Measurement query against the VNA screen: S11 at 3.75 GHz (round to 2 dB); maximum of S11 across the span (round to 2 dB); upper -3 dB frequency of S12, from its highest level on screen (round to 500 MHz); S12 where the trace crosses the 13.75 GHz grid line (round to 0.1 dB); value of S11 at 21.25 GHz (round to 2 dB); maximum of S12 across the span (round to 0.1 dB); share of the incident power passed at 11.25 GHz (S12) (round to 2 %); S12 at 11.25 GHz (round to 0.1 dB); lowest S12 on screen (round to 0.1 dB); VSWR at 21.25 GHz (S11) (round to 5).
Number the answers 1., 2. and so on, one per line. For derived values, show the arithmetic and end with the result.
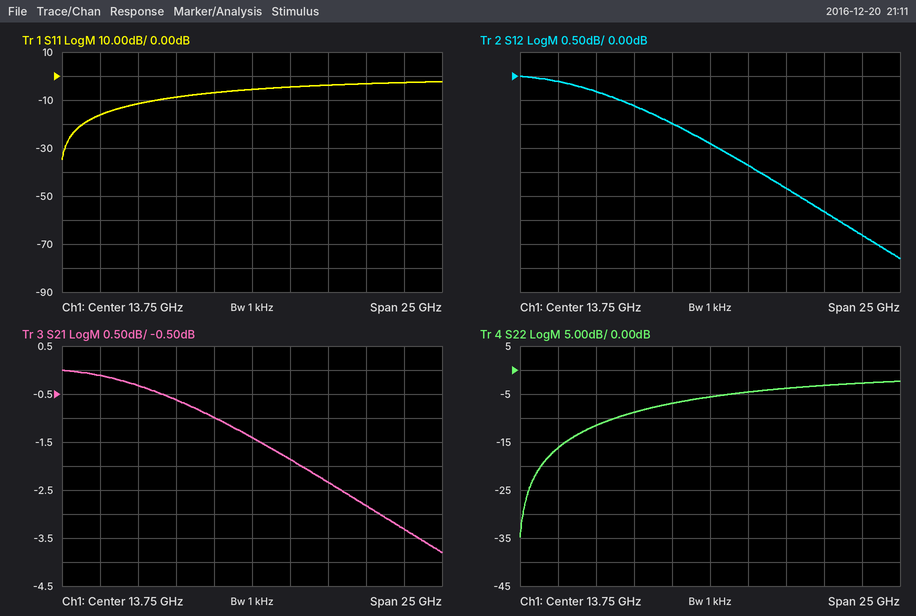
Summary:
1. -16 dB
2. -2 dB
3. 22.0 GHz
4. -1.4 dB
5. -4 dB
6. 0.0 dB
7. 10^(-1/10) ≈ 79.4 %, so 80 % to the nearest 2 %
8. -1.0 dB
9. -3.8 dB
10. |Γ| = 10^(-4/20) = 0.6310; VSWR = (1 + 0.6310)/(1 − 0.6310) ≈ 4.42, so 5 to the nearest 5
